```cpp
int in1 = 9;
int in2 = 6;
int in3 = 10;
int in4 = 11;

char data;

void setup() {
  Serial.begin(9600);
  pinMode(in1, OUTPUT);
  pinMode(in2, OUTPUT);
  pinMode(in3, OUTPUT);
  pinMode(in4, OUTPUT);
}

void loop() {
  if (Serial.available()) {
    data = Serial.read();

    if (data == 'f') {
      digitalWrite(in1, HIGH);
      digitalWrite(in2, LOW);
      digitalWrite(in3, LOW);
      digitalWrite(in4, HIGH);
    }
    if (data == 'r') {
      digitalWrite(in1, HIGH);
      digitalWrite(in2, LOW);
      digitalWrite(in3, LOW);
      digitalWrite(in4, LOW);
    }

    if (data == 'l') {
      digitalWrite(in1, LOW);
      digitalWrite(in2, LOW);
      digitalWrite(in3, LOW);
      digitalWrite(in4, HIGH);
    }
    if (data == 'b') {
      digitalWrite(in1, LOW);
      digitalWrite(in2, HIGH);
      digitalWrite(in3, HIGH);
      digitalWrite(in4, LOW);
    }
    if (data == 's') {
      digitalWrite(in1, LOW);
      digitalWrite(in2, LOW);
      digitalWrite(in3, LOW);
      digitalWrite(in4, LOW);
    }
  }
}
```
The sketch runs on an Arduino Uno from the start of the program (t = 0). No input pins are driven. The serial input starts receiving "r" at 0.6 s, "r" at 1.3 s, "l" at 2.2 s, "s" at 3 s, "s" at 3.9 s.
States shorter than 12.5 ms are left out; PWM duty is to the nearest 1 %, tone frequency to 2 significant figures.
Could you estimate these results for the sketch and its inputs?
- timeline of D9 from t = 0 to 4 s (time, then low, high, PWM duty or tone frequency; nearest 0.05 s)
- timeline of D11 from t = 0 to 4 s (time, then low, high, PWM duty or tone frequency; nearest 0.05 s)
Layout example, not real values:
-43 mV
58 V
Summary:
0 s low; 0.6 s high; 2.2 s low
0 s low; 2.2 s high; 3 s low
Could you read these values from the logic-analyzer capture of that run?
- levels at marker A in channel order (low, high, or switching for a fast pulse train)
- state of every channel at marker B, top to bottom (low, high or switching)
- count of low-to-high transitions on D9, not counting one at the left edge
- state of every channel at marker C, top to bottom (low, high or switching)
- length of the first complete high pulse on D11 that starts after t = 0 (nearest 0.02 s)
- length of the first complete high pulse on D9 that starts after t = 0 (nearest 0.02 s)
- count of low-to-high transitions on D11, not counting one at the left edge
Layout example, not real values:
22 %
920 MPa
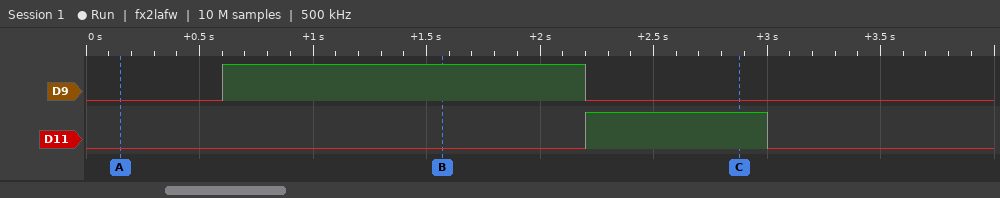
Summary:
D9 low, D11 low
D9 high, D11 low
1
D9 low, D11 high
0.80 s
1.60 s
1
